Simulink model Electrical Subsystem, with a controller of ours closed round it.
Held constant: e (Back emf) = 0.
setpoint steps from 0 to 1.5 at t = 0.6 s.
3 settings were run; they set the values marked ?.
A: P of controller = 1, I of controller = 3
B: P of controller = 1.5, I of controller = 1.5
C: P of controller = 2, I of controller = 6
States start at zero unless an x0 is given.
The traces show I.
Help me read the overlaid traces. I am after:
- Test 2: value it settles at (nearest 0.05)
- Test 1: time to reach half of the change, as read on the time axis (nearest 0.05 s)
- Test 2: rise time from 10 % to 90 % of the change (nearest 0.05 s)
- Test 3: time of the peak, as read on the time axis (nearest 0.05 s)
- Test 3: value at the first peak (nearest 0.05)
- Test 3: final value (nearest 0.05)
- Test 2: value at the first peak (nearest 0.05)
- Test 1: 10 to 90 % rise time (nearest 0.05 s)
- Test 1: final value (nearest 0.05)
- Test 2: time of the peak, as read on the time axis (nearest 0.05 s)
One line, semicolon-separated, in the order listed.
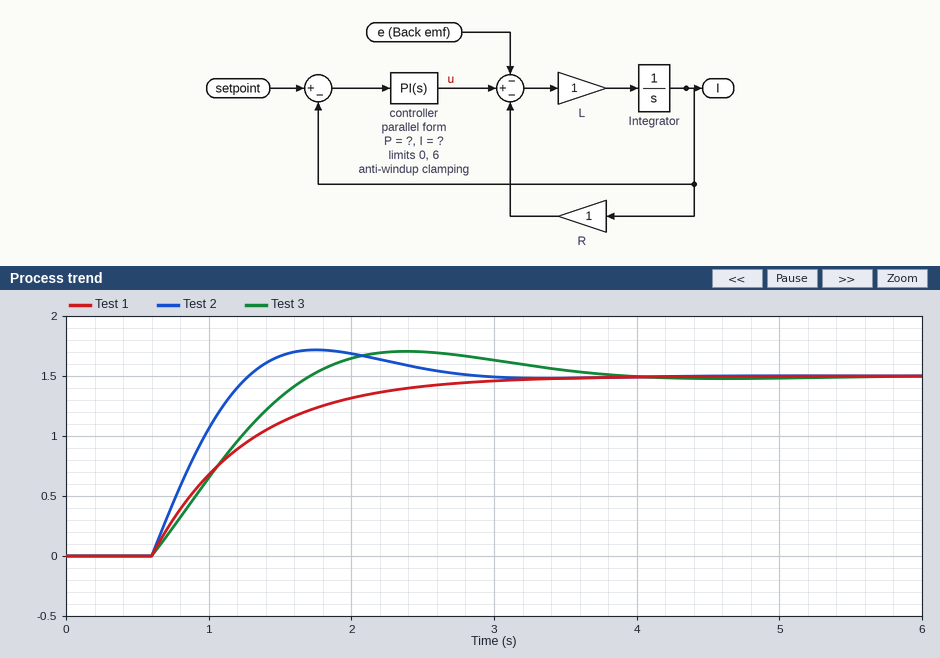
1.50; 1.05 s; 0.50 s; 2.40 s; 1.70; 1.50; 1.70; 1.45 s; 1.50; 1.75 s
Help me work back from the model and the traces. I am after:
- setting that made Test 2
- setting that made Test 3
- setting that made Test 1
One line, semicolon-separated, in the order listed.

C; A; B
